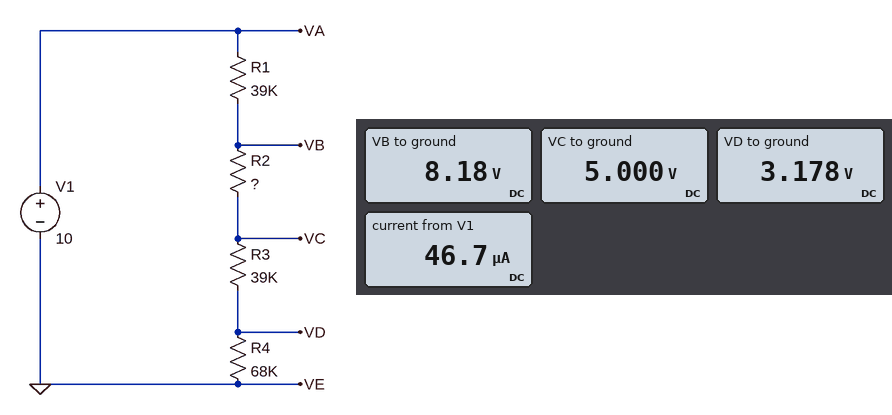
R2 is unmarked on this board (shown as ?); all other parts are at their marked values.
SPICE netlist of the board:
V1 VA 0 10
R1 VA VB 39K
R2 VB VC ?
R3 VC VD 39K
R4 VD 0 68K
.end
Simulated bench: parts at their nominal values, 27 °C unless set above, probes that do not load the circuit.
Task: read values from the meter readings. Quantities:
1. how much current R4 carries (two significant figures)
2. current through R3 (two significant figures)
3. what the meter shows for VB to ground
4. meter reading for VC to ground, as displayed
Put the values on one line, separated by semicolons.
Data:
47 µA; 47 µA; 8.18 V; 5.000 V
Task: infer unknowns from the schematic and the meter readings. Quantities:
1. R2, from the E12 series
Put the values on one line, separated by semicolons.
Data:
68 kΩ
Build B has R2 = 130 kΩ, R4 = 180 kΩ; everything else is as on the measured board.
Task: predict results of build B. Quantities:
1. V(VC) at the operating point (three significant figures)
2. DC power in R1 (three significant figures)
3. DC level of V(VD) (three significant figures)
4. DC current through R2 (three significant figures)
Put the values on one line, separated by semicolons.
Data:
5.64 V; 25.9 µW; 4.64 V; 25.8 µA
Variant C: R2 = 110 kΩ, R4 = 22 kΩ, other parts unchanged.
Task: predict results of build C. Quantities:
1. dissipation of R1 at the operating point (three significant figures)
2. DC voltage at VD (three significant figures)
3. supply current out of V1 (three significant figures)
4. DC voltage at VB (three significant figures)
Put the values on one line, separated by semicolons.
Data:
88.4 µW; 1.05 V; 47.6 µA; 8.14 V
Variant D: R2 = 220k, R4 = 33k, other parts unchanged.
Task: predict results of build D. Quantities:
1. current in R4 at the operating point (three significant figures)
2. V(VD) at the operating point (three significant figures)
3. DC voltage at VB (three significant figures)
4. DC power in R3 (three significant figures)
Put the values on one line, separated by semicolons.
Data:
30.2 µA; 997 mV; 8.82 V; 35.6 µW
